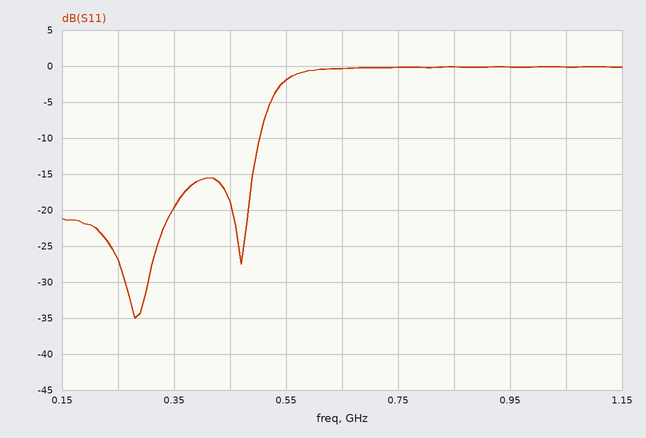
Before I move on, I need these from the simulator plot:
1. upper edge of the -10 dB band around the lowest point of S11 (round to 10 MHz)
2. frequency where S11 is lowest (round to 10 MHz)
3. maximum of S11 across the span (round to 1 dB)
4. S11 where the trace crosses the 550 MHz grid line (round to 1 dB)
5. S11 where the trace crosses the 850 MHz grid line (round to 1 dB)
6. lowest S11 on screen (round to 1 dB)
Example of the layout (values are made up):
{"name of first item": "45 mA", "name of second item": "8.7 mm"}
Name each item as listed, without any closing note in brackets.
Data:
{"upper edge of the -10 dB band around the lowest point of S11": "500 MHz", "frequency where S11 is lowest": "280 MHz", "maximum of S11 across the span": "0 dB", "S11 where the trace crosses the 550 MHz grid line": "-2 dB", "S11 where the trace crosses the 850 MHz grid line": "0 dB", "lowest S11 on screen": "-35 dB"}
